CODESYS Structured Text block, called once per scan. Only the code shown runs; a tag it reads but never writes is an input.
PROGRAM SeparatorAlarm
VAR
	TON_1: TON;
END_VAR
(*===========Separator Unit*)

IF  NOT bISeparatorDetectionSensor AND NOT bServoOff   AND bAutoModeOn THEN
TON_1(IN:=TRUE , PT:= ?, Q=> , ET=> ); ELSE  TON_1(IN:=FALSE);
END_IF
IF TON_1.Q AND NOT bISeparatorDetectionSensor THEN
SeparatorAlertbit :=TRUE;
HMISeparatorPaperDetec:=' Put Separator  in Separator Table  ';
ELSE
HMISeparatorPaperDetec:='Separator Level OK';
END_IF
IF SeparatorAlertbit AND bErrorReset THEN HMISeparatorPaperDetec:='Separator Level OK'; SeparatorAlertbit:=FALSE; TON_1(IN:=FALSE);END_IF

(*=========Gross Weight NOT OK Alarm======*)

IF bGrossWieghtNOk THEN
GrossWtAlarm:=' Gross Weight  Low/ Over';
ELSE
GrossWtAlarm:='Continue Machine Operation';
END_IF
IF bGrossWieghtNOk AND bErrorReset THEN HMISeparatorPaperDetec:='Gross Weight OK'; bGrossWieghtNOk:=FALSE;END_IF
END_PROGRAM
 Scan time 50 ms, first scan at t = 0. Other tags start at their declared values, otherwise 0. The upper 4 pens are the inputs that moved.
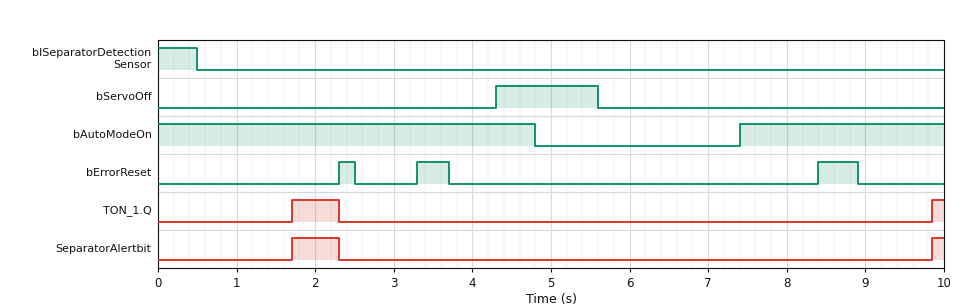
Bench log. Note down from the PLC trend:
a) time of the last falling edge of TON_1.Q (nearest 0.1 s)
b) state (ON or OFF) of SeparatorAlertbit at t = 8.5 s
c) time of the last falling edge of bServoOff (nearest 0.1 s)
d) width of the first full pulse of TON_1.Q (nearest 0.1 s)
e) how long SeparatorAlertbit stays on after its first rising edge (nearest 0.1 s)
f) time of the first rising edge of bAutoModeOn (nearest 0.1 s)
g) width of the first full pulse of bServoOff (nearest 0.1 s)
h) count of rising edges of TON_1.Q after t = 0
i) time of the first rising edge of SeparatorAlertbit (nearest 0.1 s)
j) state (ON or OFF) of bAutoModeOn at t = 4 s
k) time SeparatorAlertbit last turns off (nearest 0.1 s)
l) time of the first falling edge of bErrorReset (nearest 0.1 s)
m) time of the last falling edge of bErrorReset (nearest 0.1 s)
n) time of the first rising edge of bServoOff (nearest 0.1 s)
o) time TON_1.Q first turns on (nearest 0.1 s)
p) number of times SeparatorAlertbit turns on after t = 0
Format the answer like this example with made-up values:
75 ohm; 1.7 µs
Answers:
2.3 s; OFF; 5.6 s; 0.6 s; 0.6 s; 7.4 s; 1.3 s; 2; 1.7 s; ON; 2.3 s; 2.5 s; 8.9 s; 4.3 s; 1.7 s; 2
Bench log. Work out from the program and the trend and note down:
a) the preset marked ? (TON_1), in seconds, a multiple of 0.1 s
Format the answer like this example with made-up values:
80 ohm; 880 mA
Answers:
1.2 s
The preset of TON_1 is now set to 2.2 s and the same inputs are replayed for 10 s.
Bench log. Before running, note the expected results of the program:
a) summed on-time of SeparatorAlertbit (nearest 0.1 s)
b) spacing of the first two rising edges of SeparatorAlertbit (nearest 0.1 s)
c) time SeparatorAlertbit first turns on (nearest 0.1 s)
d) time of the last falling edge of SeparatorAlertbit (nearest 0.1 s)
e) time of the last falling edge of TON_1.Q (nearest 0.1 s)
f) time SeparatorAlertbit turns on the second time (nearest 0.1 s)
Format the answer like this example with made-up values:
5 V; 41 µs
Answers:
1.0 s; 6.9 s; 2.7 s; 3.3 s; 3.3 s; 9.6 s
